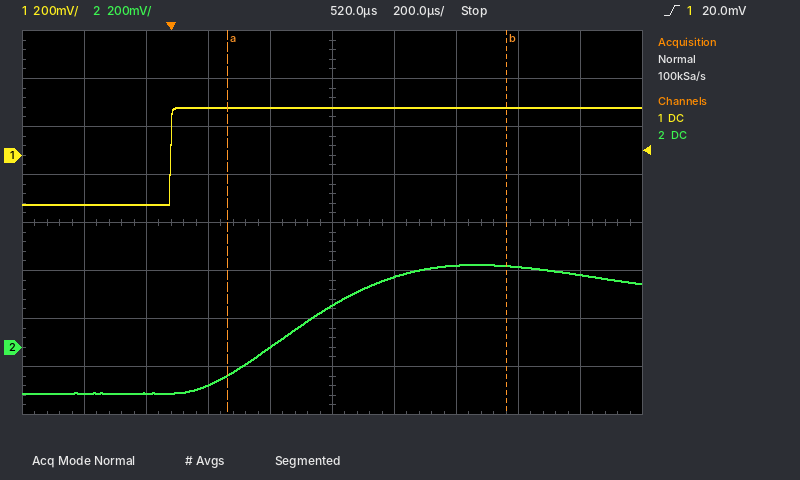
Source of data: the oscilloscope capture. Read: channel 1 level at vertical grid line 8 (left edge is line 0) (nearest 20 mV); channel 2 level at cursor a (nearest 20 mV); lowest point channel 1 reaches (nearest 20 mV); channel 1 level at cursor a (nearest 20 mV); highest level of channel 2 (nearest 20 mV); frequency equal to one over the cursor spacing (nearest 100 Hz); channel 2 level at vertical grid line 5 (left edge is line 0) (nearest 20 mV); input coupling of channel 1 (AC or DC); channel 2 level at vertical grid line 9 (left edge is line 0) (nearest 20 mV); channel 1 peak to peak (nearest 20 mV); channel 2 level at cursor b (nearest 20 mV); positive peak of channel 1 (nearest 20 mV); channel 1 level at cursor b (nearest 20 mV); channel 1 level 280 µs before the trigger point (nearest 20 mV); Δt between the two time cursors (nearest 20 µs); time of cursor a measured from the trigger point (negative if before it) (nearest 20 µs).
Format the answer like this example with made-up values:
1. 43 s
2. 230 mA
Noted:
1. 200 mV
2. -120 mV
3. -200 mV
4. 200 mV
5. 340 mV
6. 1.1 kHz
7. 180 mV
8. DC
9. 300 mV
10. 400 mV
11. 340 mV
12. 200 mV
13. 200 mV
14. -200 mV
15. 900 µs
16. +180 µs
